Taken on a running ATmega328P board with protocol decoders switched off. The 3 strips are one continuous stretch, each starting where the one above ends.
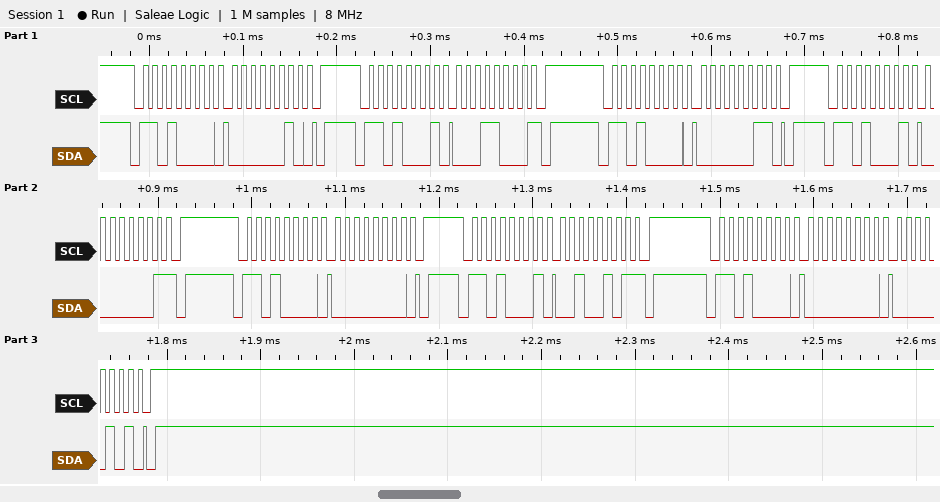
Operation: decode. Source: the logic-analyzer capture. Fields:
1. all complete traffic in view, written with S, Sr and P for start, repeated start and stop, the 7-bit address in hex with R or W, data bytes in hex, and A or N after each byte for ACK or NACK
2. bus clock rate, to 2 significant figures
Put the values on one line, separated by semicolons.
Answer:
S 68W A 02 A P S 68R A 18 N P S 68W A 03 A P S 68R A 01 N P S 68W A 00 A P S 68R A 25 N P S 68W A 00 A 05 A P; 100 kHz
